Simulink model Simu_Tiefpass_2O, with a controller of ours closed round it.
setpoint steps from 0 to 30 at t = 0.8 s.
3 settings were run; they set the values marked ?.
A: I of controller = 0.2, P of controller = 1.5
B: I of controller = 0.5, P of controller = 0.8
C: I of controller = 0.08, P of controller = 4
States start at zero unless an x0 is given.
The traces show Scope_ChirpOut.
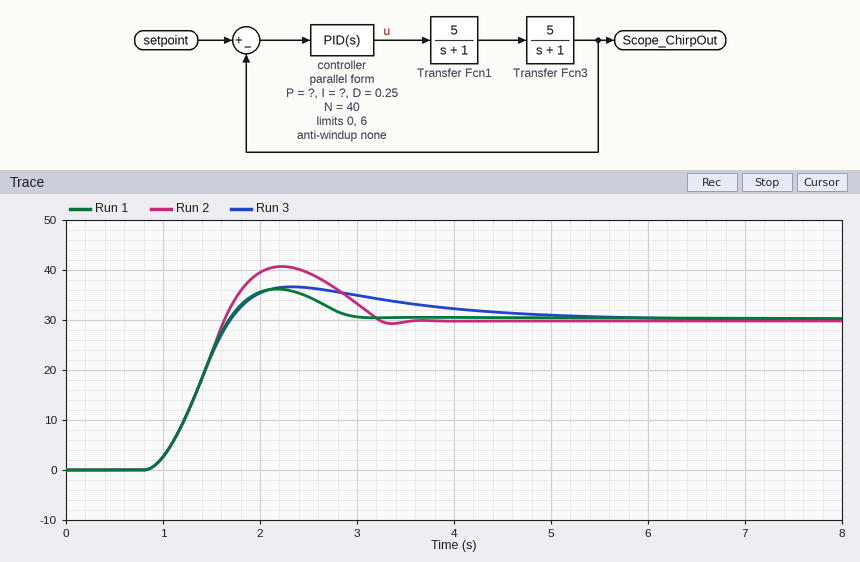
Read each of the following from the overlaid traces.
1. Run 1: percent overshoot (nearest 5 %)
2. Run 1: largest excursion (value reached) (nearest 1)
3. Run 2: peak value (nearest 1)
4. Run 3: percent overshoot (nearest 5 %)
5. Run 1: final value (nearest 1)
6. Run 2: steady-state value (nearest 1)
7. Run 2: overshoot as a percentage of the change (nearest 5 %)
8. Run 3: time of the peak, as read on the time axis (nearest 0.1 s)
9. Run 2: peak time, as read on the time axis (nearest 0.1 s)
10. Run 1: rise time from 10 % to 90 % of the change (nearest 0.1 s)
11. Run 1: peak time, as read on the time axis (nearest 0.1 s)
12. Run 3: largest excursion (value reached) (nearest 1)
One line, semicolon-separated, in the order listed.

20 %; 36; 41; 20 %; 30; 30; 35 %; 2.3 s; 2.2 s; 0.6 s; 2.2 s; 37
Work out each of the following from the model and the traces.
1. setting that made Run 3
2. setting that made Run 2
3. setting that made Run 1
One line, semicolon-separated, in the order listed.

B; C; A
